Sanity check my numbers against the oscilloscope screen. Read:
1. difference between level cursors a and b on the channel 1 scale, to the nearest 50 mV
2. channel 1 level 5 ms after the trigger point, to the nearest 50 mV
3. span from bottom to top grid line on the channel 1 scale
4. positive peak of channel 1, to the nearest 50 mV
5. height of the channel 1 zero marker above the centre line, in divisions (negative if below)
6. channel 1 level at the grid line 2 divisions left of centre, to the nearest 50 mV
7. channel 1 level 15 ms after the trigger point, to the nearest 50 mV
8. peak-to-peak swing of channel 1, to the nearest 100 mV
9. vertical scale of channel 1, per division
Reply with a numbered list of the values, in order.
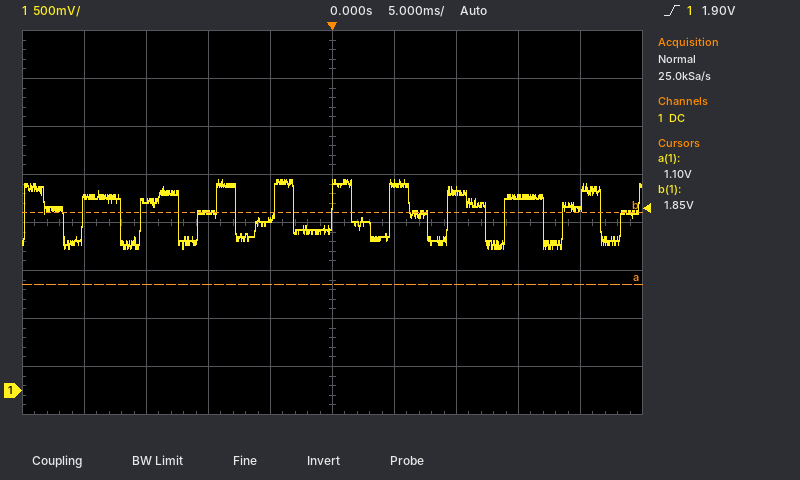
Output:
1. 750 mV
2. 2.15 V
3. 4 V
4. 2.20 V
5. -3.5 div
6. 1.85 V
7. 2.00 V
8. 700 mV
9. 500 mV
